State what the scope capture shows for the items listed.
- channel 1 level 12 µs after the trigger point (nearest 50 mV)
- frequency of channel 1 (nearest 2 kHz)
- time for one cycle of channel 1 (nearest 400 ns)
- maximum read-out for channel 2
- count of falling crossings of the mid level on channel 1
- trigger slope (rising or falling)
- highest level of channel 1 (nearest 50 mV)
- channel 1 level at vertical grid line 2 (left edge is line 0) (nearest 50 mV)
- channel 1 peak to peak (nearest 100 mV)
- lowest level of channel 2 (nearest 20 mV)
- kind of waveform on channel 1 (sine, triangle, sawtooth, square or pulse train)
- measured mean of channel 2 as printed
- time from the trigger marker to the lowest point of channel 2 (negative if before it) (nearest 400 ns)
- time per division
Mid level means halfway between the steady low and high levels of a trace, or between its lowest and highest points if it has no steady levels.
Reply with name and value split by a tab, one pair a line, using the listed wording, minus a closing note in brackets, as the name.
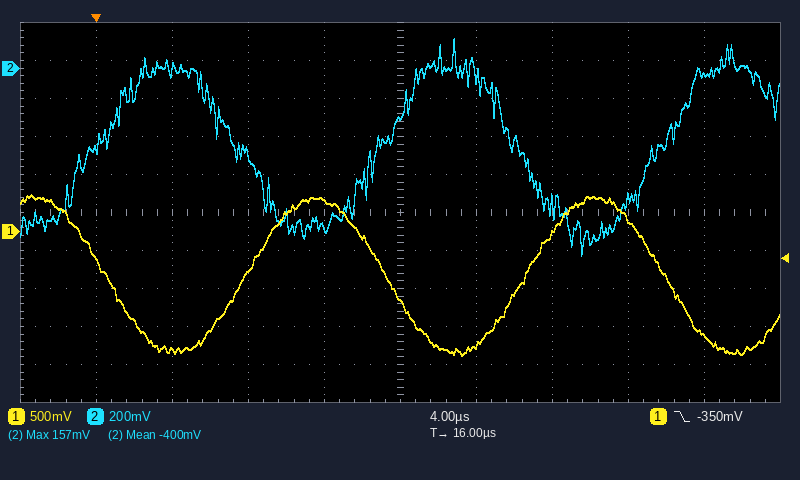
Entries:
channel 1 level 12 µs after the trigger point	400 mV
frequency of channel 1	68 kHz
time for one cycle of channel 1	14.8 µs
maximum read-out for channel 2	157 mV
count of falling crossings of the mid level on channel 1	3
trigger slope	falling
highest level of channel 1	500 mV
channel 1 level at vertical grid line 2 (left edge is line 0)	-1.55 V
channel 1 peak to peak	2.10 V
lowest level of channel 2	-980 mV
kind of waveform on channel 1	sine
measured mean of channel 2 as printed	-400 mV
time from the trigger marker to the lowest point of channel 2 (negative if before it)	+25.6 µs
time per division	4 µs
